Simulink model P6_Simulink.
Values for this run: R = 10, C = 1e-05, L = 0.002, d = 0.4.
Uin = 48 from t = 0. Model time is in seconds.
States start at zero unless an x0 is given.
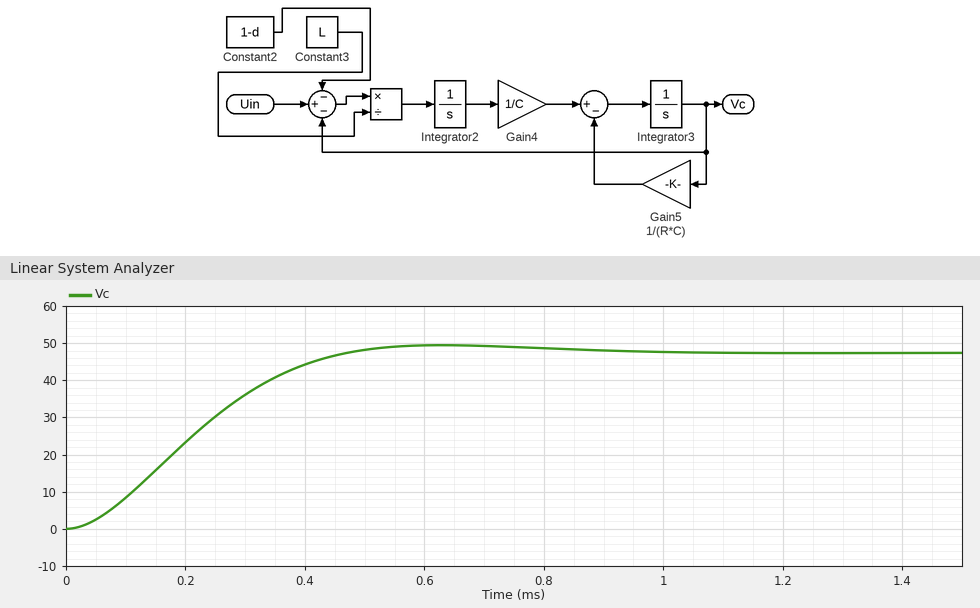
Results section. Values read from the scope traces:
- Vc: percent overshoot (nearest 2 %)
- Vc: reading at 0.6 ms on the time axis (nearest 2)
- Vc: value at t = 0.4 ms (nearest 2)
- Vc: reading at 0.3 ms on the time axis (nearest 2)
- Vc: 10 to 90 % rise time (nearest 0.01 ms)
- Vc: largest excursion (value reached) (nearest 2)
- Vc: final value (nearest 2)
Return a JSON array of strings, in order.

["4 %", "50", "44", "36", "0.30 ms", "50", "48"]
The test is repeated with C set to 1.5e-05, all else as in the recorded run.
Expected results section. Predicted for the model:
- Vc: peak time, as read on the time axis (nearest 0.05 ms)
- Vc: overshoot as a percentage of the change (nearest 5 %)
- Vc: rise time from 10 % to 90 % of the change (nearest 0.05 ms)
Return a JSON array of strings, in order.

["0.65 ms", "10 %", "0.30 ms"]
